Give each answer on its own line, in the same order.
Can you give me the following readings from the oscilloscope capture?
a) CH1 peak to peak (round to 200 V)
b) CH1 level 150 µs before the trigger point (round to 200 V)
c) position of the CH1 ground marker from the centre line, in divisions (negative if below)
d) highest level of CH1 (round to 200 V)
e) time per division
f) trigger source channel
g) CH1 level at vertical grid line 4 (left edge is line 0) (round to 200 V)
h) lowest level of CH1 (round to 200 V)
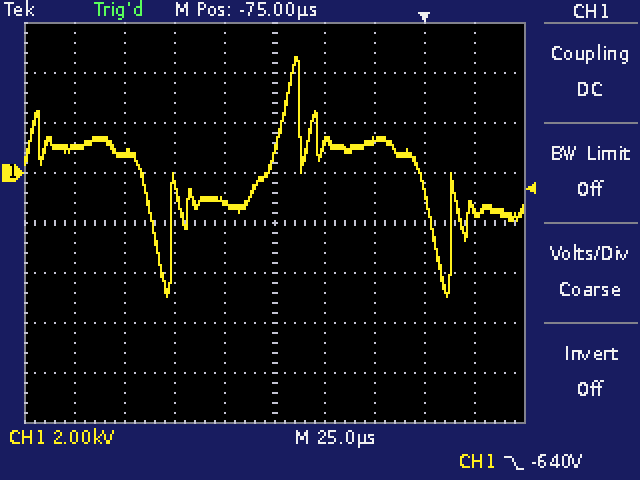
9.6 kV
800 V
+1.0 div
4.6 kV
25 µs
CH1
-1.2 kV
-5.0 kV
